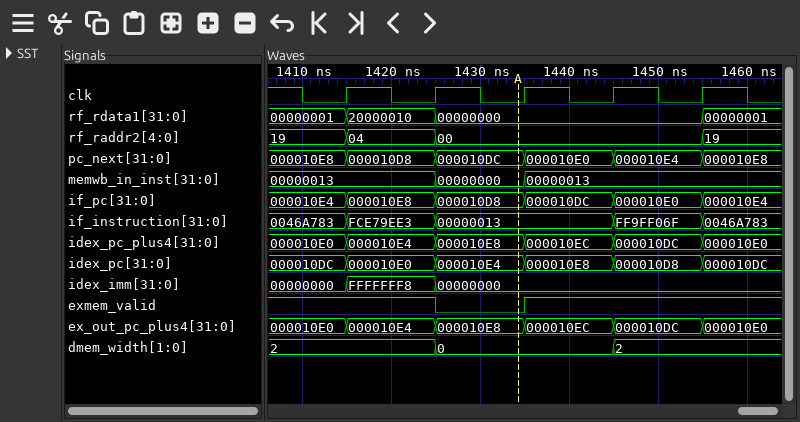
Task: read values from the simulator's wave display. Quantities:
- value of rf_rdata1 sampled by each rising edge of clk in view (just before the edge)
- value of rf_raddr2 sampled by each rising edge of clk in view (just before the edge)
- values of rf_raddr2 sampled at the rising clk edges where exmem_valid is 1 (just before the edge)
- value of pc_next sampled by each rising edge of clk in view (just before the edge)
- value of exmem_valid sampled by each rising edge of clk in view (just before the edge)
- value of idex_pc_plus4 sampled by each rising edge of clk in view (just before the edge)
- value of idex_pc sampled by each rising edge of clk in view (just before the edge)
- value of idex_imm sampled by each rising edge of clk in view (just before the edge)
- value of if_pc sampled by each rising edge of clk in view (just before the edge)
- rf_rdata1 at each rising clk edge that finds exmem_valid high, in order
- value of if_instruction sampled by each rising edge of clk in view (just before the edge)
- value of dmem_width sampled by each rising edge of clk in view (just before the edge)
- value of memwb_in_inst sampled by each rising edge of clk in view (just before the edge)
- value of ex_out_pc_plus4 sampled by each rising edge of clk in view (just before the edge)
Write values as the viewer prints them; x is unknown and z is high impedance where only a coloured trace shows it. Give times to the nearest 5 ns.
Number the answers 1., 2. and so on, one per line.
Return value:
1. 00000001, 20000010, 00000000, 00000000, 00000000
2. 19, 04, 00, 00, 00
3. 19, 04, 00, 00
4. 000010E8, 000010D8, 000010DC, 000010E0, 000010E4
5. 1 1 0 1 1
6. 000010E0, 000010E4, 000010E8, 000010EC, 000010DC
7. 000010DC, 000010E0, 000010E4, 000010E8, 000010D8
8. 00000000, FFFFFFF8, 00000000, 00000000, 00000000
9. 000010E4, 000010E8, 000010D8, 000010DC, 000010E0
10. 00000001, 20000010, 00000000, 00000000
11. 0046A783, FCE79EE3, 00000013, 00000013, FF9FF06F
12. 2, 2, 0, 0, 2
13. 00000013, 00000013, 00000000, 00000013, 00000013
14. 000010E0, 000010E4, 000010E8, 000010EC, 000010DC
